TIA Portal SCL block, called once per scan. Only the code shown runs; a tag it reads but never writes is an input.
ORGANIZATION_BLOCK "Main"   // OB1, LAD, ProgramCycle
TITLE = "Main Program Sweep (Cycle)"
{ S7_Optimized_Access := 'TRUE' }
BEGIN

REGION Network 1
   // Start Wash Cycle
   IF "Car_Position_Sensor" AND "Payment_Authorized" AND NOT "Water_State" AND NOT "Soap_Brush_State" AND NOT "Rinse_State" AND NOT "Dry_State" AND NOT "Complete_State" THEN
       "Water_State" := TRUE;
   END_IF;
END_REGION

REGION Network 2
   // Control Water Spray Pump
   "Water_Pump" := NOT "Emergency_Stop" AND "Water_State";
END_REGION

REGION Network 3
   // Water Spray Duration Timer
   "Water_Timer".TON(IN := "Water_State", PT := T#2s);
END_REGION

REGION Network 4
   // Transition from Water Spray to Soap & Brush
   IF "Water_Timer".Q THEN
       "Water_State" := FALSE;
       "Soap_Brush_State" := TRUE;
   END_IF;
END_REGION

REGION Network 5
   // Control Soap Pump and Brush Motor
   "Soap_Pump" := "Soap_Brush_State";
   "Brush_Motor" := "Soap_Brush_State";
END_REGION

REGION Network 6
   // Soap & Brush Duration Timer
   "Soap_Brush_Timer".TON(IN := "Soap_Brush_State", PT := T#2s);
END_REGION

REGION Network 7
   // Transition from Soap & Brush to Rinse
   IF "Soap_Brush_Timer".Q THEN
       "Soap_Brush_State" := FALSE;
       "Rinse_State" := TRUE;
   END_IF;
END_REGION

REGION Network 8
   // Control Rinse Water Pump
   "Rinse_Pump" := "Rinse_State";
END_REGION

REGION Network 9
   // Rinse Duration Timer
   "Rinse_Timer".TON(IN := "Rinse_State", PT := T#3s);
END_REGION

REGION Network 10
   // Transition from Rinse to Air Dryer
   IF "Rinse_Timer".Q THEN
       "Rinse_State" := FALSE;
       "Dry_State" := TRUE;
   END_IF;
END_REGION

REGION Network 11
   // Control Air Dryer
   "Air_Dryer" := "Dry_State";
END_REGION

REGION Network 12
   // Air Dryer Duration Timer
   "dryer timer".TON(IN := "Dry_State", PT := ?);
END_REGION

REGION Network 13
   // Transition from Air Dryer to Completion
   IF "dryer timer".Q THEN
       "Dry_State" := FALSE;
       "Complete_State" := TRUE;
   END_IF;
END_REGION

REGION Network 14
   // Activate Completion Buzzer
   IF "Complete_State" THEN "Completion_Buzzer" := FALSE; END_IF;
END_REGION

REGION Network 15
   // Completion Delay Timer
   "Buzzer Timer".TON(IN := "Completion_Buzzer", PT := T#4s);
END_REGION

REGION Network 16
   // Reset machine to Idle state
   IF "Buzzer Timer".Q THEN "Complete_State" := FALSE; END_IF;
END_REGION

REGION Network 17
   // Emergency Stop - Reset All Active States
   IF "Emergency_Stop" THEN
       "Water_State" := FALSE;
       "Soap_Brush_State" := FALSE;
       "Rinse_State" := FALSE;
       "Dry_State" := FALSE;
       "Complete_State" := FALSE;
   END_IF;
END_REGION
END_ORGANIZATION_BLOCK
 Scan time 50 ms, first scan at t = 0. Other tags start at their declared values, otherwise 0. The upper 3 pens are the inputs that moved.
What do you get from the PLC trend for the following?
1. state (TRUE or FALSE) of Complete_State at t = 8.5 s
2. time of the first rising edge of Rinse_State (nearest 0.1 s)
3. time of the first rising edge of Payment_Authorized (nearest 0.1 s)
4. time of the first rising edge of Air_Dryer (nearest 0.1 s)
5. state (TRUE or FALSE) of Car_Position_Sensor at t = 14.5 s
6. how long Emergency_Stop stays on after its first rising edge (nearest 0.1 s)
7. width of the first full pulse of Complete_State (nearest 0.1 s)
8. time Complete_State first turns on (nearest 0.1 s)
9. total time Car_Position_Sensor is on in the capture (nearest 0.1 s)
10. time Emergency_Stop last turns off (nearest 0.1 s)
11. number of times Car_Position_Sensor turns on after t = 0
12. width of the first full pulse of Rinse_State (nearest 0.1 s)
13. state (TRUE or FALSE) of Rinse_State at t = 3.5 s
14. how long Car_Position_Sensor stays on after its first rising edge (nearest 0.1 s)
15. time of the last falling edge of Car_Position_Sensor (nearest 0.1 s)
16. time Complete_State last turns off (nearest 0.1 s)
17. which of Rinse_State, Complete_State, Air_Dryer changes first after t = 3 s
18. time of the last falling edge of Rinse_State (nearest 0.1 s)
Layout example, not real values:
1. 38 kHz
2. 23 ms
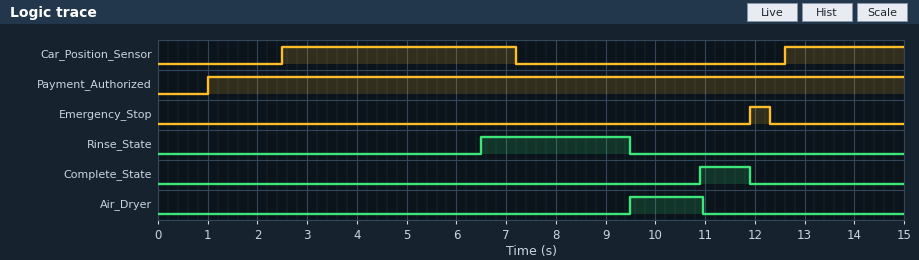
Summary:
1. FALSE
2. 6.5 s
3. 1.0 s
4. 9.5 s
5. TRUE
6. 0.4 s
7. 1.0 s
8. 10.9 s
9. 7.1 s
10. 12.3 s
11. 2
12. 3.0 s
13. FALSE
14. 4.7 s
15. 7.2 s
16. 11.9 s
17. Rinse_State
18. 9.5 s
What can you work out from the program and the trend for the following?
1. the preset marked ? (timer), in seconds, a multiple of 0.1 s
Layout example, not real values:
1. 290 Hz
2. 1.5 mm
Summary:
1. 1.4 s
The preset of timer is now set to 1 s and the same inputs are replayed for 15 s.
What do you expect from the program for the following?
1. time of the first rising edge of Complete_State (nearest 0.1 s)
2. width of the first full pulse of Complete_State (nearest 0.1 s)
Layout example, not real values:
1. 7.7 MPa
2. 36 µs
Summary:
1. 10.5 s
2. 1.4 s
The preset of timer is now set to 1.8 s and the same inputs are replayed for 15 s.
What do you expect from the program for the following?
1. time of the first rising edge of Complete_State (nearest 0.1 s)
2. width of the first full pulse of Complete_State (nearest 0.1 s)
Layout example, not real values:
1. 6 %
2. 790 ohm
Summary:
1. 11.3 s
2. 0.6 s
